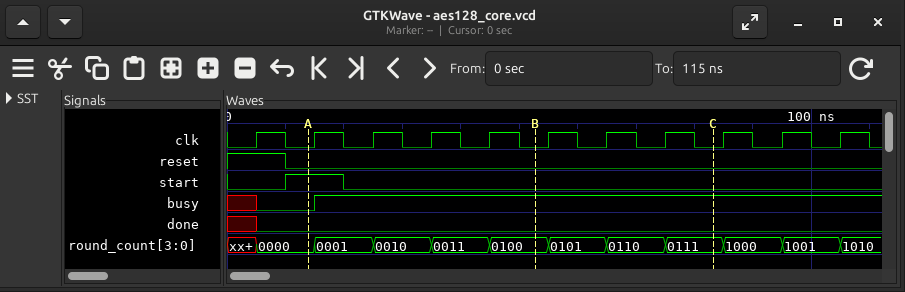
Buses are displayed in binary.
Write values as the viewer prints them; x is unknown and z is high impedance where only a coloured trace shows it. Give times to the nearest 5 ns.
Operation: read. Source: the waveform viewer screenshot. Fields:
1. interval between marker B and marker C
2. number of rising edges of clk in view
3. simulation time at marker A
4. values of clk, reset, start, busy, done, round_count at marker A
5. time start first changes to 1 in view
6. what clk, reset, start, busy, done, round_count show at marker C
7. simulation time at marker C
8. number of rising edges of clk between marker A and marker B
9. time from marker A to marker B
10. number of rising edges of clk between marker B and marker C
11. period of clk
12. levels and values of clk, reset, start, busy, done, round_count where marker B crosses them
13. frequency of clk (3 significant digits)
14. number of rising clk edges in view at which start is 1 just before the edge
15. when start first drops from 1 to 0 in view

30 ns
11
15 ns
clk=0, reset=0, start=1, busy=0, done=0, round_count=0000
10 ns
clk=0, reset=0, start=0, busy=1, done=0, round_count=0111
85 ns
4
40 ns
3
10 ns
clk=0, reset=0, start=0, busy=1, done=0, round_count=0100
100 MHz
1
20 ns
